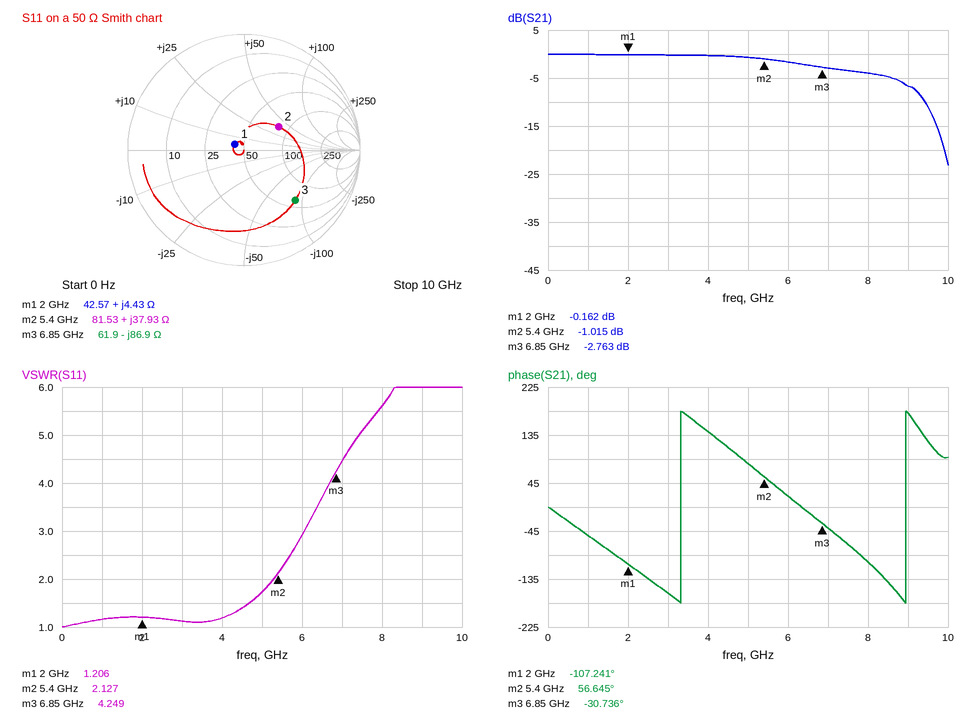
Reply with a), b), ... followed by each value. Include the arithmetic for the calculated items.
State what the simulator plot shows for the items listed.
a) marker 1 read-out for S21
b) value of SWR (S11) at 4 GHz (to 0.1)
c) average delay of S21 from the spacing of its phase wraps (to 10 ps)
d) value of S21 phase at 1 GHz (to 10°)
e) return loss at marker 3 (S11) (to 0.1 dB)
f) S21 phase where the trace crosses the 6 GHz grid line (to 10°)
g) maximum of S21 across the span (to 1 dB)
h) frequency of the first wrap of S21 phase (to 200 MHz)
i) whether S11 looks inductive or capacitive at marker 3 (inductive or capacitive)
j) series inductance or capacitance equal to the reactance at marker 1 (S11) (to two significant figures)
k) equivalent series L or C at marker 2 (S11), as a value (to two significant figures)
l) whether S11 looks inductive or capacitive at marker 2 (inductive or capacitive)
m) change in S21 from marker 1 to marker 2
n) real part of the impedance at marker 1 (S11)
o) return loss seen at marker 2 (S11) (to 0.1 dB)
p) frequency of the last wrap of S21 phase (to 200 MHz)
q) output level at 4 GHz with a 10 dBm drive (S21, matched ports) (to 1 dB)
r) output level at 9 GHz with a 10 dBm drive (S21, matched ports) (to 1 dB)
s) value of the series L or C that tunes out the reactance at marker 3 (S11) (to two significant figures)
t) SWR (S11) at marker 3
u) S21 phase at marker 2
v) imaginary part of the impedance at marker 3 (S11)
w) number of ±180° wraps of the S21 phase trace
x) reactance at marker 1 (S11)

a) -0.162 dB
b) 1.2
c) 1 cycle / (9.0 GHz − 3.4 GHz) ≈ 179 ps, so 180 ps to the nearest 10 ps
d) -50°
e) 4.2 dB
f) 20°
g) 0 dB
h) 3.4 GHz
i) capacitive
j) L = 4.43 Ω/(2π × 2 GHz) ≈ 353 pH, so 350 pH to two significant figures
k) L = 37.93 Ω/(2π × 5.4 GHz) ≈ 1.1 nH
l) inductive
m) -1.015 − (-0.162) = -0.853 dB
n) 42.57 Ω
o) 8.9 dB
p) 9.0 GHz
q) 10 dBm + (0 dB) = 10 dBm
r) 10 dBm + (-7 dB) = 3 dBm
s) L = 86.9 Ω/(2π × 6.85 GHz) ≈ 2.0 nH
t) 4.249
u) 56.645°
v) -86.9 Ω
w) 2
x) +4.43 Ω
